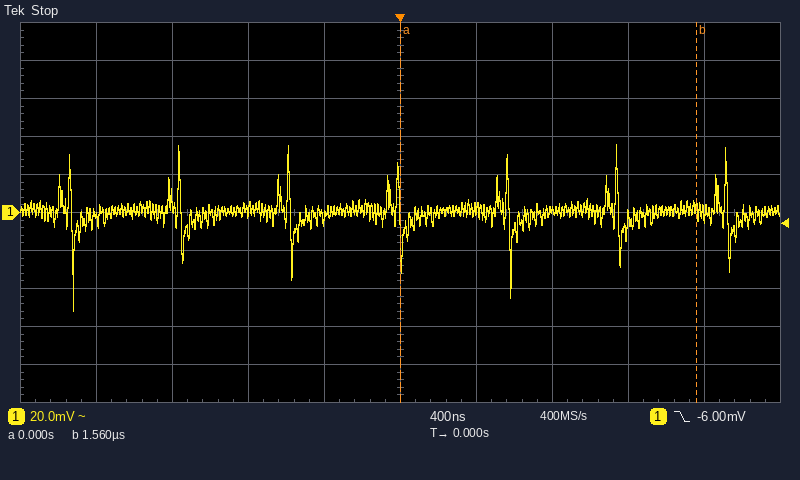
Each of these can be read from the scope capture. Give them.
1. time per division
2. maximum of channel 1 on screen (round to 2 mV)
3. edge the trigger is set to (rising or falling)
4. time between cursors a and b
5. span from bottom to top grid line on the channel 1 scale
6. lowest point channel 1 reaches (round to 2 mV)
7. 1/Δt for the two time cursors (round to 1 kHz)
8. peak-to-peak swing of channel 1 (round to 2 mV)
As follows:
400 ns
36 mV
falling
1.56 µs
200 mV
-52 mV
641 kHz
88 mV
